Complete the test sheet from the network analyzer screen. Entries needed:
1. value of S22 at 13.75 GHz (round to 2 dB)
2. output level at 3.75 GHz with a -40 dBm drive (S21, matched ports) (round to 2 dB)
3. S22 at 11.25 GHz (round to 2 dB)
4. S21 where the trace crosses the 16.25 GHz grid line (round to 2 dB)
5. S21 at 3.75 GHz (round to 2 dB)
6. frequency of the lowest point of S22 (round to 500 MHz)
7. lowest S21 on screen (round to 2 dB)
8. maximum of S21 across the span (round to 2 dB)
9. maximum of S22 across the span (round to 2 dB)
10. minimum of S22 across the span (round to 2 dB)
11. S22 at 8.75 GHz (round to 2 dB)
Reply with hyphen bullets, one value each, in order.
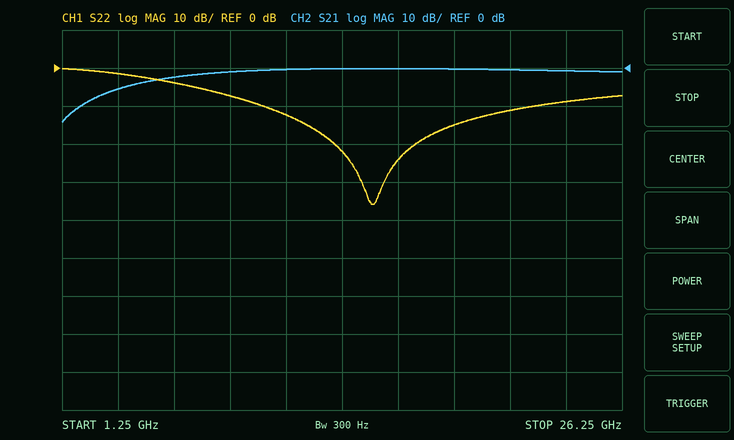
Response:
- -22 dB
- -46 dBm
- -12 dB
- 0 dB
- -6 dB
- 15.0 GHz
- -14 dB
- 0 dB
- 0 dB
- -36 dB
- -8 dB
